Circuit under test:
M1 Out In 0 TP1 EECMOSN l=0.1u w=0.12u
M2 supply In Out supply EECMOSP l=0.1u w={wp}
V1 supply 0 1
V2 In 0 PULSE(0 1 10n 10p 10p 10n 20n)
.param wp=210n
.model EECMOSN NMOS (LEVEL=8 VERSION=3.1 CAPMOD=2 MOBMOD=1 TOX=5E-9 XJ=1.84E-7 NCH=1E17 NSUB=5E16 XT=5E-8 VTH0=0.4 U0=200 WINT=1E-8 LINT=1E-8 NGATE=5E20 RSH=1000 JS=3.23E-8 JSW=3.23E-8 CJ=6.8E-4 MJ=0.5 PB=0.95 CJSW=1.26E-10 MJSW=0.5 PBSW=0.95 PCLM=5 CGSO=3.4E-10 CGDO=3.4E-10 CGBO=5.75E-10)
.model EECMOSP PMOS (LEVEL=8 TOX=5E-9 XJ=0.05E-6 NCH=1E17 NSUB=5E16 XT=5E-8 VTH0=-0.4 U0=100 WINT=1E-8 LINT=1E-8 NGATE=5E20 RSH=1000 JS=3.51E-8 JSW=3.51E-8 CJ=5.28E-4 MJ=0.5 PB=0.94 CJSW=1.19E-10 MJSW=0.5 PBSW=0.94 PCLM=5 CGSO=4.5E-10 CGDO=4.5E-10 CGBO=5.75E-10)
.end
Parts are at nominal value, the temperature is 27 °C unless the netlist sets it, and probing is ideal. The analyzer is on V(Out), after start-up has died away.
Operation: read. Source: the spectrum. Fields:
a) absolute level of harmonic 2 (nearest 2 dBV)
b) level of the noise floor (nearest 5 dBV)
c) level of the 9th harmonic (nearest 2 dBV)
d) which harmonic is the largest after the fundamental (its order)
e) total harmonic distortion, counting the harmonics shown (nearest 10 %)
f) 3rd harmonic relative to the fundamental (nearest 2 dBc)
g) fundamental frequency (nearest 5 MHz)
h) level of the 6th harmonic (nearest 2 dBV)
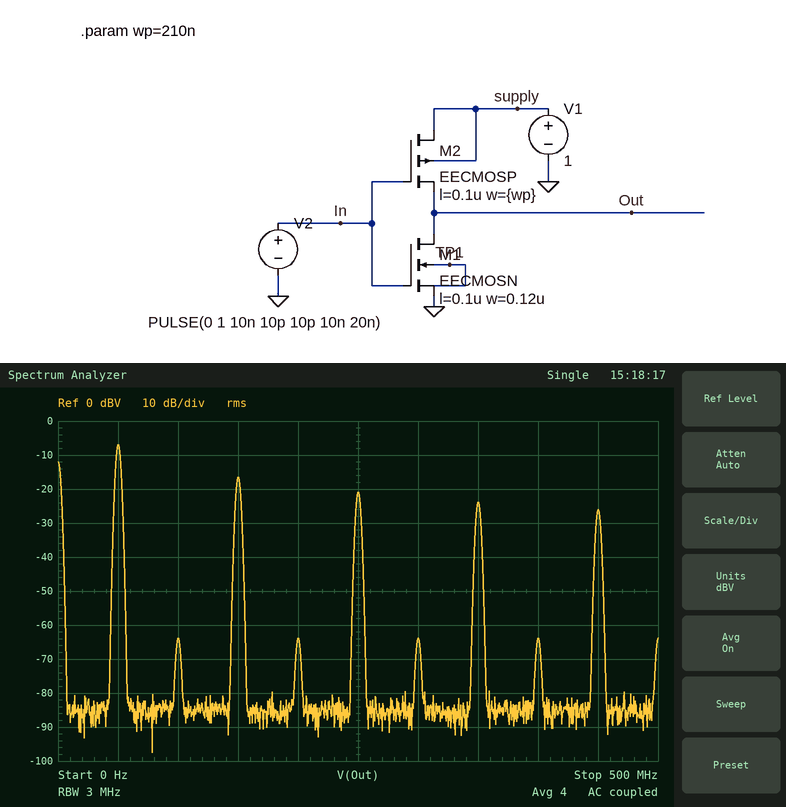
-64 dBV
-85 dBV
-26 dBV
3
40 %
-10 dBc
50 MHz
-64 dBV
